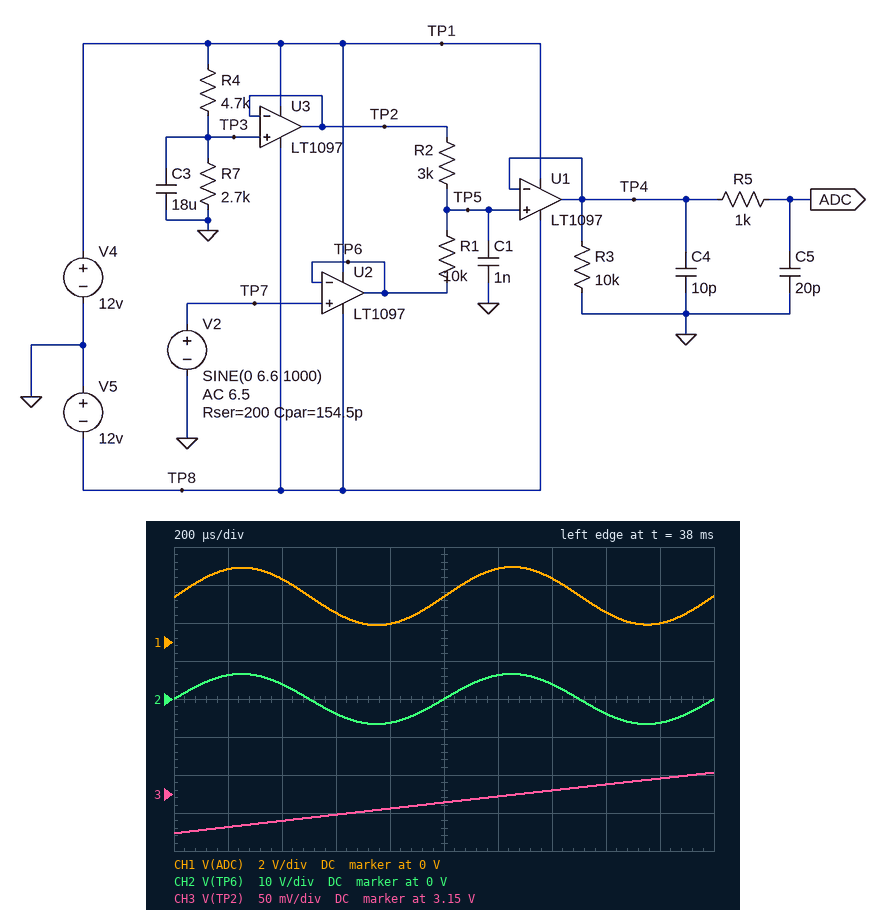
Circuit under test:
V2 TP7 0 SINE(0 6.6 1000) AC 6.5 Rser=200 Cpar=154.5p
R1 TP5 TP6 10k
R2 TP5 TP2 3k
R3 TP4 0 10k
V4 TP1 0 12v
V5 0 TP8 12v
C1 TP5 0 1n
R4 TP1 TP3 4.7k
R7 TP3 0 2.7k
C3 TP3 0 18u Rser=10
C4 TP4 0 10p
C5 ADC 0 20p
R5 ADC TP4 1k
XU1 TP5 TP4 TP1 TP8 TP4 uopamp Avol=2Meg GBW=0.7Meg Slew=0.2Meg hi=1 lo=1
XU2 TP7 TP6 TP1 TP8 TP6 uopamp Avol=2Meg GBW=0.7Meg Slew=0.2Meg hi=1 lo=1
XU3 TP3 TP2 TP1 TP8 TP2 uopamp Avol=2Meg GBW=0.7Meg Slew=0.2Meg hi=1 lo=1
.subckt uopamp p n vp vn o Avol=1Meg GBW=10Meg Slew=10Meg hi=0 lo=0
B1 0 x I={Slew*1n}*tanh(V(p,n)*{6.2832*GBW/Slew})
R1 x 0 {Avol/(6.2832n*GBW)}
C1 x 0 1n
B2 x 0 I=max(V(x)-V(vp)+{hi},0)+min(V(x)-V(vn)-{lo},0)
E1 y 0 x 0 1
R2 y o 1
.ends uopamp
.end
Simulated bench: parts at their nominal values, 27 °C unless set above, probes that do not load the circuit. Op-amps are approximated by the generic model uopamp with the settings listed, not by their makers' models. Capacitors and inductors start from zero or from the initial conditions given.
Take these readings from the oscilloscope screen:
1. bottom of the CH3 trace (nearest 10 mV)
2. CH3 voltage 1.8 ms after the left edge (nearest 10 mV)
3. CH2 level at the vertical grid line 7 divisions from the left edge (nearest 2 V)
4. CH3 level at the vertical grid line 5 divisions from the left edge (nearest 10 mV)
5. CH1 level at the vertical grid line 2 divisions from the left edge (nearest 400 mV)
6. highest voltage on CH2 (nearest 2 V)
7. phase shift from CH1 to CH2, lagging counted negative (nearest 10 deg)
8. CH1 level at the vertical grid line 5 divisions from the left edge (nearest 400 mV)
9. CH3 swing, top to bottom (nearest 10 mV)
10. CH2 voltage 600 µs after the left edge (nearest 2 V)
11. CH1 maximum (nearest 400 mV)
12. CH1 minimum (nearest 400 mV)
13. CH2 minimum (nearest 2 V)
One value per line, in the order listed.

3.10 V
3.17 V
4 V
3.14 V
3.2 V
6 V
0 deg
2.4 V
80 mV
-4 V
4.0 V
800 mV
-6 V
